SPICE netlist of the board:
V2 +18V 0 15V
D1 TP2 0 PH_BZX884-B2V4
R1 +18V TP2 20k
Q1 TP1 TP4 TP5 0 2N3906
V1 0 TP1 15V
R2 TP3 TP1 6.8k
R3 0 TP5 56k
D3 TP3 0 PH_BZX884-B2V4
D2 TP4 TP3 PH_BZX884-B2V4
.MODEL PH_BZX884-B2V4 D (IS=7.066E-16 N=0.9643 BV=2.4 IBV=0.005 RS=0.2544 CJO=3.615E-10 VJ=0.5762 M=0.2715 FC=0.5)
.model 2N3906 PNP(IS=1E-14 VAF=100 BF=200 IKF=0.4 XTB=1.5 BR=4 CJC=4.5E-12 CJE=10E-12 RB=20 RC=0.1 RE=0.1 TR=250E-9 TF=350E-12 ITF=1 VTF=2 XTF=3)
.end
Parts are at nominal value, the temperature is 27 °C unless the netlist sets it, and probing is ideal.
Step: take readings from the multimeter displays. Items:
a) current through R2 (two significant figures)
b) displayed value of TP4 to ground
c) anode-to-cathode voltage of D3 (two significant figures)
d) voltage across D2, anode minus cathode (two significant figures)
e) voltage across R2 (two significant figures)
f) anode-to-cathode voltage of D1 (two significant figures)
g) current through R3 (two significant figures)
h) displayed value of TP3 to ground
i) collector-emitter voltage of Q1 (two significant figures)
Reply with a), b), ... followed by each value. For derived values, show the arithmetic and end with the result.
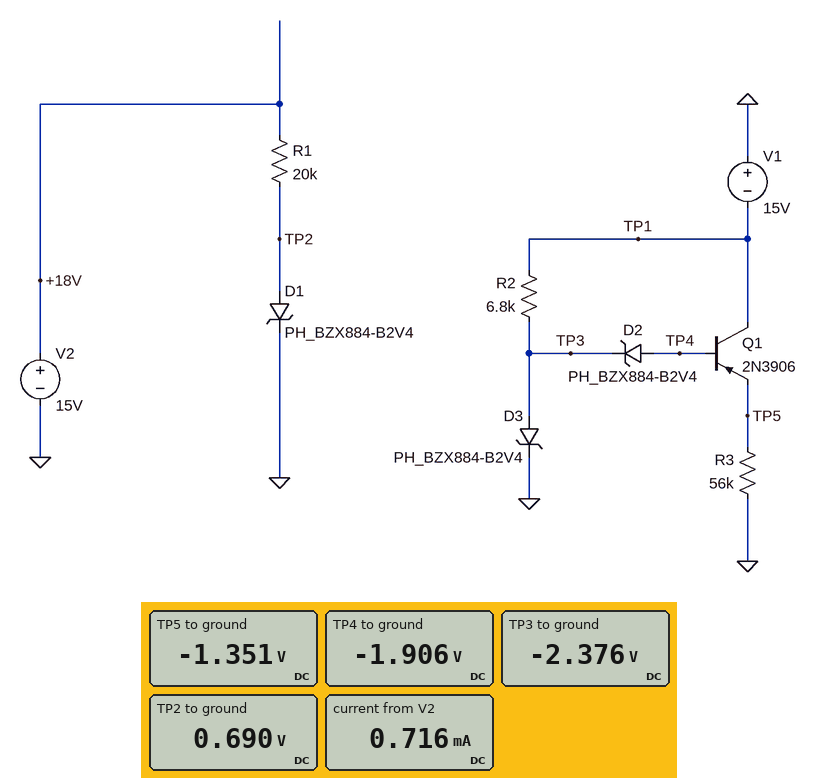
a) (-2.376 V - (-15 V)) / 6.8 kΩ = 1.9 mA
b) -1.906 V
c) -2.376 V = -2.4 V
d) -1.906 V - (-2.376 V) = 470 mV
e) -2.376 V - (-15 V) = 13 V
f) 690 mV = 690 mV
g) (0 V - (-1.351 V)) / 56 kΩ = 24 µA
h) -2.376 V
i) -15 V - (-1.351 V) = -14 V
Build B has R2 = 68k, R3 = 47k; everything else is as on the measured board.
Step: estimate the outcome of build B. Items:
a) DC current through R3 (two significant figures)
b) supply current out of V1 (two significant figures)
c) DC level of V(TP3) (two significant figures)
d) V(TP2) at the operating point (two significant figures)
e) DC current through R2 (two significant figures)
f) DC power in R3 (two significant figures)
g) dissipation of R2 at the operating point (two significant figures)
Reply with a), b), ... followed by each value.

a) 27 µA
b) 210 µA
c) -2.3 V
d) 690 mV
e) 190 µA
f) 35 µW
g) 2.4 mW
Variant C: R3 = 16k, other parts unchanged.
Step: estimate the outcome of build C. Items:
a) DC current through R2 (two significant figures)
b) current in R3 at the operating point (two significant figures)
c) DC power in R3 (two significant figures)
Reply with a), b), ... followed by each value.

a) 1.9 mA
b) 81 µA
c) 100 µW
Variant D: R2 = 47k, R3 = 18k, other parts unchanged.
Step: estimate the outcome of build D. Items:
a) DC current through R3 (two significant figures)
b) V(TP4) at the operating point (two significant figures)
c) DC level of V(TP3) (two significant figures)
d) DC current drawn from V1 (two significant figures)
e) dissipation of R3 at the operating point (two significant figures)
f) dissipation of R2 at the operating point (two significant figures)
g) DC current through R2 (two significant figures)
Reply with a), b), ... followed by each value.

a) 69 µA
b) -1.8 V
c) -2.3 V
d) 340 µA
e) 87 µW
f) 3.4 mW
g) 270 µA
